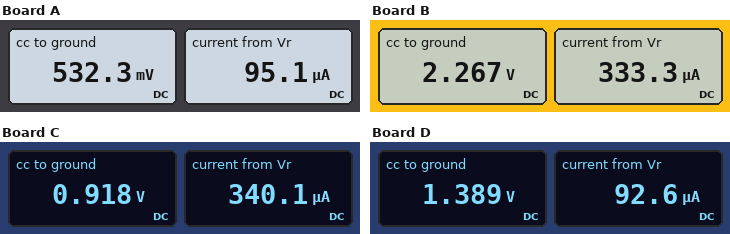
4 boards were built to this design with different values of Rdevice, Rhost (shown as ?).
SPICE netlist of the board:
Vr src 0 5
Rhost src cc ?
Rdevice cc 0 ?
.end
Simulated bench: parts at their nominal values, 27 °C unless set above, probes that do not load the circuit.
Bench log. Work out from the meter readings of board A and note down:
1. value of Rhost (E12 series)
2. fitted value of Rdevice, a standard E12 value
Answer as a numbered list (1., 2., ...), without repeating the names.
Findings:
1. 47 kΩ
2. 5.6 kΩ
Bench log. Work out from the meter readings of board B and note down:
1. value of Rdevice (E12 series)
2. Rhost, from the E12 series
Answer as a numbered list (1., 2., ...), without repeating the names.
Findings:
1. 6.8 kΩ
2. 8.2 kΩ
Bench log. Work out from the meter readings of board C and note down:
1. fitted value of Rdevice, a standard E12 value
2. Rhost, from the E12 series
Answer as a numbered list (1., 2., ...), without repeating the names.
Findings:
1. 2.7 kΩ
2. 12 kΩ
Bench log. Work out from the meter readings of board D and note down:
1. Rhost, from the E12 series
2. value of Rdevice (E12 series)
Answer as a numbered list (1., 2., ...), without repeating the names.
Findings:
1. 39 kΩ
2. 15 kΩ
